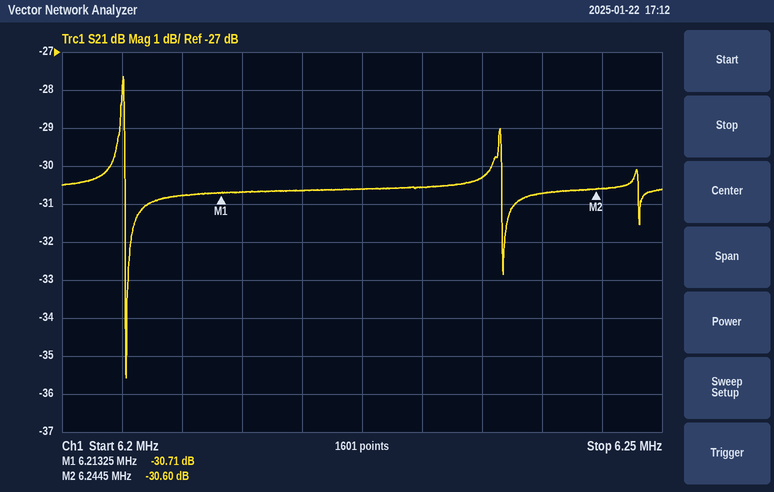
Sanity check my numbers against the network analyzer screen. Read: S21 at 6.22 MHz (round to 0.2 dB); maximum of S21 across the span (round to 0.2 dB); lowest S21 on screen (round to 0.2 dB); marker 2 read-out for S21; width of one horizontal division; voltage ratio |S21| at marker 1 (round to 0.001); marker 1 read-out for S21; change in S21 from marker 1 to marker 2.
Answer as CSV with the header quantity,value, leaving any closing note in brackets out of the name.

quantity,value
S21 at 6.22 MHz,-30.6 dB
maximum of S21 across the span,-27.6 dB
lowest S21 on screen,-35.6 dB
marker 2 read-out for S21,-30.60 dB
width of one horizontal division,5 kHz
voltage ratio |S21| at marker 1,0.029
marker 1 read-out for S21,-30.71 dB
change in S21 from marker 1 to marker 2,0.11 dB
